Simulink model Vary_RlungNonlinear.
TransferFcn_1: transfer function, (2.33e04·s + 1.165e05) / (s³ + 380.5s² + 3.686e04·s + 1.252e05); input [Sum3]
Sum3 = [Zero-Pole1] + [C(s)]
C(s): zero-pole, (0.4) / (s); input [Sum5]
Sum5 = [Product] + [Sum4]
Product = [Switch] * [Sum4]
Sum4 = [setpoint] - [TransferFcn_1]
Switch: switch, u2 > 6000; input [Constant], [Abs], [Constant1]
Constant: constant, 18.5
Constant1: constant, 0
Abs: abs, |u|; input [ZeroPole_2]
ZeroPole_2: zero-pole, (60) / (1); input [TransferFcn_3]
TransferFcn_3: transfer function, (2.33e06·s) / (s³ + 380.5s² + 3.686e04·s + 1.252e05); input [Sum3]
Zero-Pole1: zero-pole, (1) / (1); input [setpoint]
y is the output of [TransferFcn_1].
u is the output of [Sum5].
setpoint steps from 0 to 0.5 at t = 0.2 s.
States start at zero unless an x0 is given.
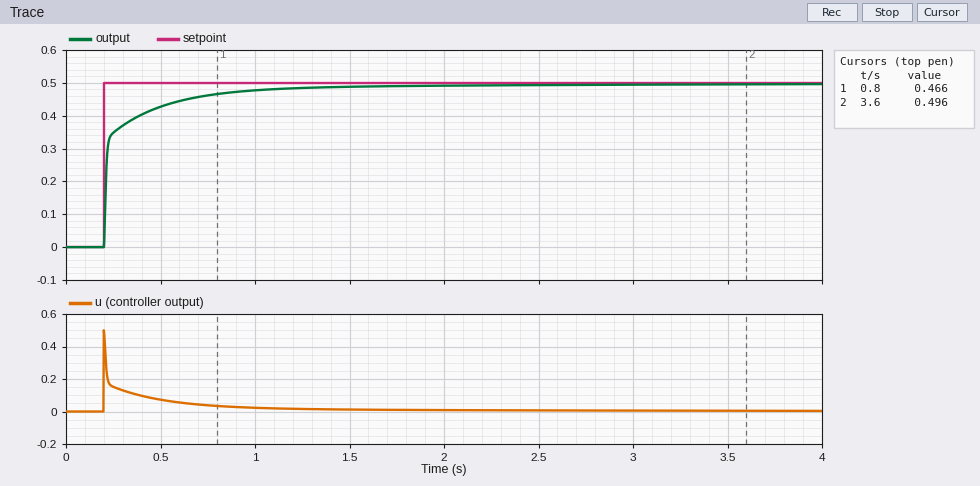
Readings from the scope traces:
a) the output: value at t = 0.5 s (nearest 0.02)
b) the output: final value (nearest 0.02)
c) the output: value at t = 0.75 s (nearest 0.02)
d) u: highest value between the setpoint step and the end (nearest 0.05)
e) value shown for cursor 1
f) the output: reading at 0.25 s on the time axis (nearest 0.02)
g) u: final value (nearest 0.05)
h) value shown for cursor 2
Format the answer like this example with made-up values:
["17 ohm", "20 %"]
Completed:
["0.42", "0.50", "0.46", "0.50", "0.466", "0.34", "0.00", "0.496"]
